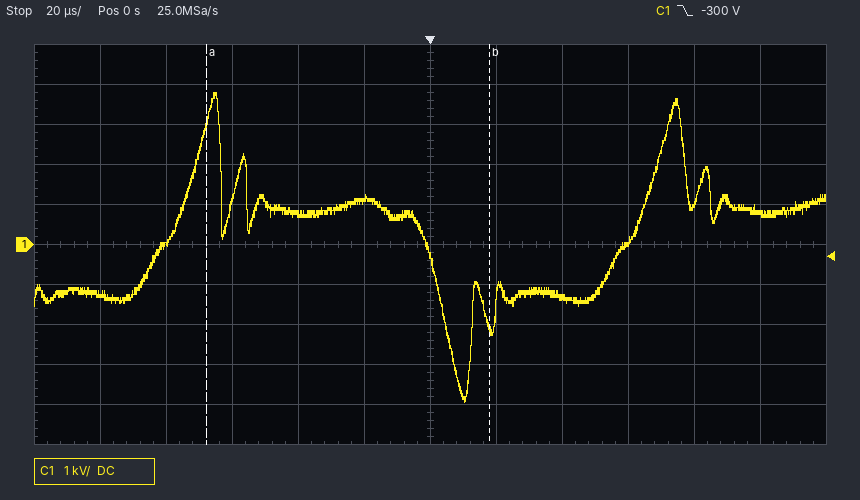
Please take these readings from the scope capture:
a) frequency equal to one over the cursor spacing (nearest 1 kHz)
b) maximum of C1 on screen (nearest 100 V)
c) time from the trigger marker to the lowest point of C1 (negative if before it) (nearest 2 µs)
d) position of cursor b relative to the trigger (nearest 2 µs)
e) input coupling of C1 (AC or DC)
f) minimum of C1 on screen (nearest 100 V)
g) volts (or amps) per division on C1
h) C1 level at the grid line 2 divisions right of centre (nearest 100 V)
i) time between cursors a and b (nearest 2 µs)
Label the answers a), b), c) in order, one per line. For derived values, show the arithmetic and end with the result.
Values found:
a) 1 / 86 µs ≈ 12 kHz
b) 3.8 kV
c) +10 µs
d) +18 µs
e) DC
f) -4.0 kV
g) 1 kV
h) -1.3 kV
i) 86 µs
